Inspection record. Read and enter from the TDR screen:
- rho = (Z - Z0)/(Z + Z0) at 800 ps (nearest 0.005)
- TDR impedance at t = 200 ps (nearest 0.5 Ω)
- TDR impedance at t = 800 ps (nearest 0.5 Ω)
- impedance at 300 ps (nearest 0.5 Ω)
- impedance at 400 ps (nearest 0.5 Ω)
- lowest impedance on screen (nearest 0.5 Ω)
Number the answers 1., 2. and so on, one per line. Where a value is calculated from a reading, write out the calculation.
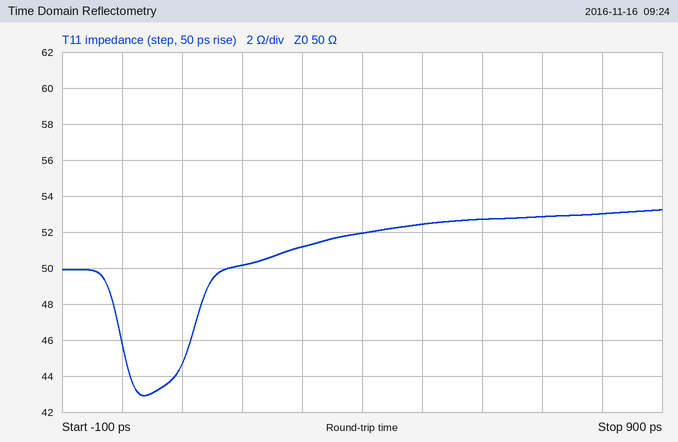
1. (53 − 50)/(53 + 50) ≈ +0.0291, so +0.030 to the nearest 0.005
2. 50.0 Ω
3. 53.0 Ω
4. 51.0 Ω
5. 52.0 Ω
6. 43.0 Ω
